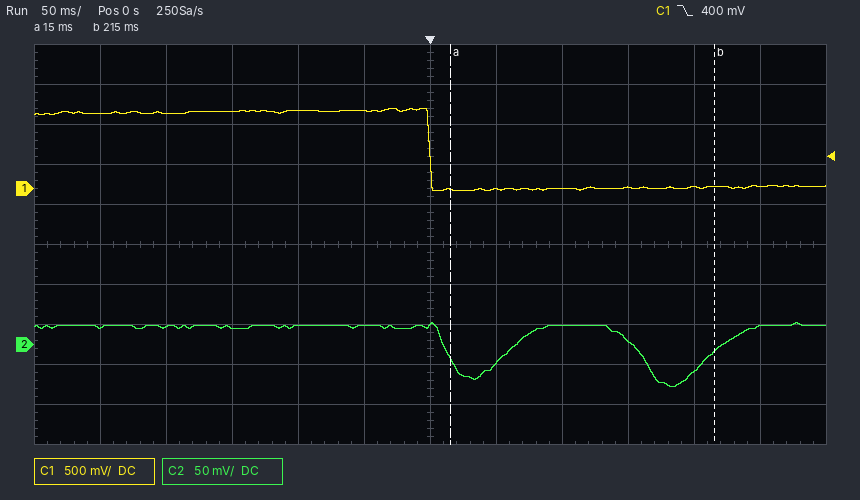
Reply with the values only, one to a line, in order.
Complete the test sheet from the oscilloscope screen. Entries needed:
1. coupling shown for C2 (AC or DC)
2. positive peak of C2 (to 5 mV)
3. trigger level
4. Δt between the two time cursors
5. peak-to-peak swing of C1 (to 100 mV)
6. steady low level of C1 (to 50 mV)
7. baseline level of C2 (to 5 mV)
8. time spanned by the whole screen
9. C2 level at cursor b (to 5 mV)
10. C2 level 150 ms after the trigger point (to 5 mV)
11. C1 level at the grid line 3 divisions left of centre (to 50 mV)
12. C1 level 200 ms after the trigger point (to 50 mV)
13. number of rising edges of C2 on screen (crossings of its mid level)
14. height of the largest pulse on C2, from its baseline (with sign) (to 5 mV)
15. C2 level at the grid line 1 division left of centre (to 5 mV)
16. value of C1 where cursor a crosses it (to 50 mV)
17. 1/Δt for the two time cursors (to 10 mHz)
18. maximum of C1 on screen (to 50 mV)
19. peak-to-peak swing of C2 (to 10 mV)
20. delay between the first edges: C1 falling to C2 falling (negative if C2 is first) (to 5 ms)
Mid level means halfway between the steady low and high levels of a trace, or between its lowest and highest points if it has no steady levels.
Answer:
DC
30 mV
400 mV
200 ms
1.00 V
0 mV
25 mV
600 ms
-10 mV
5 mV
950 mV
0 mV
2
-75 mV
25 mV
0 mV
5.00 Hz
1.00 V
80 mV
+15 ms
